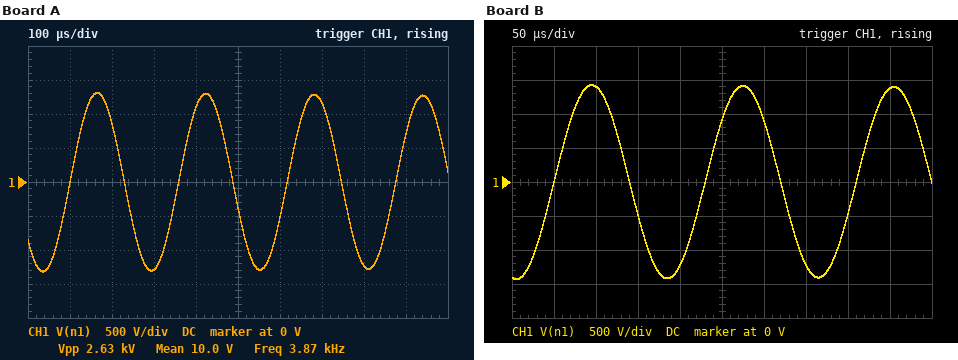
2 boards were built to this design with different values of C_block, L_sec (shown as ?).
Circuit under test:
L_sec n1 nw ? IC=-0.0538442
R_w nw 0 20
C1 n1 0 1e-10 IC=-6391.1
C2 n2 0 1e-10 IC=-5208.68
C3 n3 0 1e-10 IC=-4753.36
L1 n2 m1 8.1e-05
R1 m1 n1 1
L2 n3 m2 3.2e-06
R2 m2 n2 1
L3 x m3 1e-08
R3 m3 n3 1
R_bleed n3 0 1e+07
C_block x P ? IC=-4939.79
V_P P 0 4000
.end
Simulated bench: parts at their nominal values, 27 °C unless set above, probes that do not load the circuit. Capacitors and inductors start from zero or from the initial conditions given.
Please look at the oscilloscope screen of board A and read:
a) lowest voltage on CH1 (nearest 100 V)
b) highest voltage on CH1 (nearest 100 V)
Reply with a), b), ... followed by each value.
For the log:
a) -1.3 kV
b) 1.3 kV
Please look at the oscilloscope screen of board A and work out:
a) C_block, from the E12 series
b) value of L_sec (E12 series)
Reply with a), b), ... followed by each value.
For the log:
a) 3.3 nF
b) 470 mH
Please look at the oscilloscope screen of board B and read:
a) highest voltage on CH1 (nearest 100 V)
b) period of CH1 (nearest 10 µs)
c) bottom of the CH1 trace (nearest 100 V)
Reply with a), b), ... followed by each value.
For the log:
a) 1.4 kV
b) 180 µs
c) -1.4 kV
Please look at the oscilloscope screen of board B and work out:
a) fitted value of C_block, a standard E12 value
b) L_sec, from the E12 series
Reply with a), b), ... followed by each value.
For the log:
a) 1.8 nF
b) 390 mH
